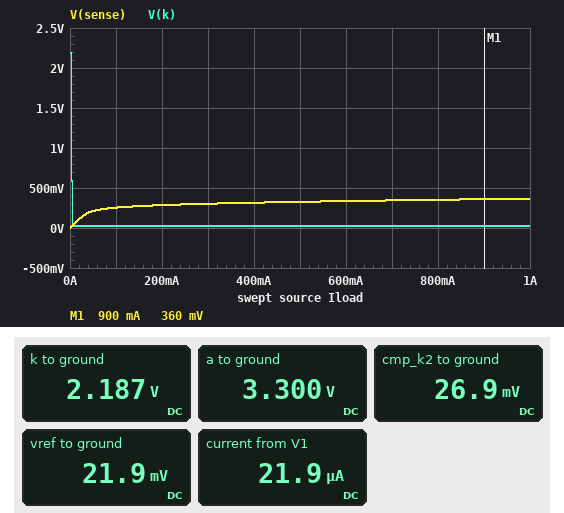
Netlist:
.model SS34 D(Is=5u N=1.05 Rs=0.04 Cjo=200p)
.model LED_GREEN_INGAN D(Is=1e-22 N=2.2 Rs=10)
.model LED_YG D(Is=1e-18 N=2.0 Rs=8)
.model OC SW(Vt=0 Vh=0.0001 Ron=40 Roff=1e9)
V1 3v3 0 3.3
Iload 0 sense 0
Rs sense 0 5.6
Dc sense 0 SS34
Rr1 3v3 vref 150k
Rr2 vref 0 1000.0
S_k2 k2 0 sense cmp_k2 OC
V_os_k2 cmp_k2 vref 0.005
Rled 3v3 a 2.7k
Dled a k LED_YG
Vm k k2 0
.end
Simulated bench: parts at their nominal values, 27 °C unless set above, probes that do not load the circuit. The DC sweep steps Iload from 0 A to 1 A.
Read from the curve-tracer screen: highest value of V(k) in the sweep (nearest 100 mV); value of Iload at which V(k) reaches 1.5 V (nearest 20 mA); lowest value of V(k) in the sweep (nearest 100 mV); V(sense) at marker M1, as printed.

2.2 V
0 A
0 V
360 mV
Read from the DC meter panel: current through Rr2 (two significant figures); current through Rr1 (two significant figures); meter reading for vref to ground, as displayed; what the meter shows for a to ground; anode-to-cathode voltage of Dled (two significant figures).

22 µA
22 µA
21.9 mV
3.300 V
1.1 V
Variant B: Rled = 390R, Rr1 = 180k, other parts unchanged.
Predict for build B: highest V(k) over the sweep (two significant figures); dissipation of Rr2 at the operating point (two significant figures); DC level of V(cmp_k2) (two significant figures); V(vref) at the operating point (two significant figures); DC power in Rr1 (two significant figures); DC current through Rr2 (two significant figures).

2.2 V
330 nW
23 mV
18 mV
60 µW
18 µA
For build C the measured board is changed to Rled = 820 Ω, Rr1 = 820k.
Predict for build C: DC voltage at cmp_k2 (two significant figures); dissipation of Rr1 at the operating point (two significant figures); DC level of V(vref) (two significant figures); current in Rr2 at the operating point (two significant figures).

9.0 mV
13 µW
4.0 mV
4.0 µA
